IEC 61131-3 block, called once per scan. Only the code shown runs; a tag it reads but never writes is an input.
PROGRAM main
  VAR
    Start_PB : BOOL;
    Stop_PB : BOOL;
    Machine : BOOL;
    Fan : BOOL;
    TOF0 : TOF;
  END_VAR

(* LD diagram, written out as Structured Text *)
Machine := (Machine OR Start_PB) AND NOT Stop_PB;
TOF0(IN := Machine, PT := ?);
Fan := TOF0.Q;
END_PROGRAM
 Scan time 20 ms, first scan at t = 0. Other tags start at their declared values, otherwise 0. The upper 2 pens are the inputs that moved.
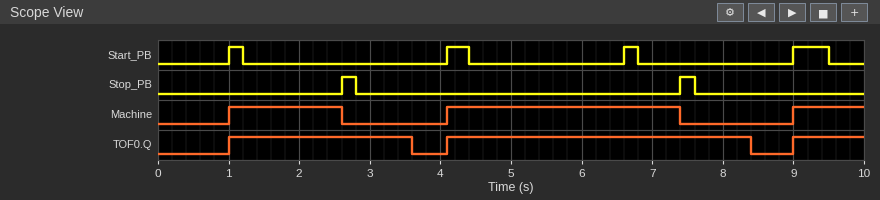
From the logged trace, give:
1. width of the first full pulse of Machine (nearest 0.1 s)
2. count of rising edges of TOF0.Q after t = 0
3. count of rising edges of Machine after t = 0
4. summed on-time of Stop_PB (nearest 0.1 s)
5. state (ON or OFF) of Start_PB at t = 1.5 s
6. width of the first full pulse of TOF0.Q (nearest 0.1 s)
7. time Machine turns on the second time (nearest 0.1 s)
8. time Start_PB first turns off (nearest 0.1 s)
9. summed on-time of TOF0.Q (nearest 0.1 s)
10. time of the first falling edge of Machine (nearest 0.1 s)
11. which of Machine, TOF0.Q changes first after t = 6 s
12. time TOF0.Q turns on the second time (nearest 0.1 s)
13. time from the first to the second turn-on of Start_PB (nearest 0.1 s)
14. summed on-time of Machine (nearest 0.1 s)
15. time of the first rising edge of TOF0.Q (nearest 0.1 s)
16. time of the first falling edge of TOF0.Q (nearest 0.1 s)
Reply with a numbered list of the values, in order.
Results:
1. 1.6 s
2. 3
3. 3
4. 0.4 s
5. OFF
6. 2.6 s
7. 4.1 s
8. 1.2 s
9. 7.9 s
10. 2.6 s
11. Machine
12. 4.1 s
13. 3.1 s
14. 5.9 s
15. 1.0 s
16. 3.6 s
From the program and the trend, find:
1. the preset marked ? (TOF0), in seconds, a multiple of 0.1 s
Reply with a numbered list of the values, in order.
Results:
1. 1.0 s
